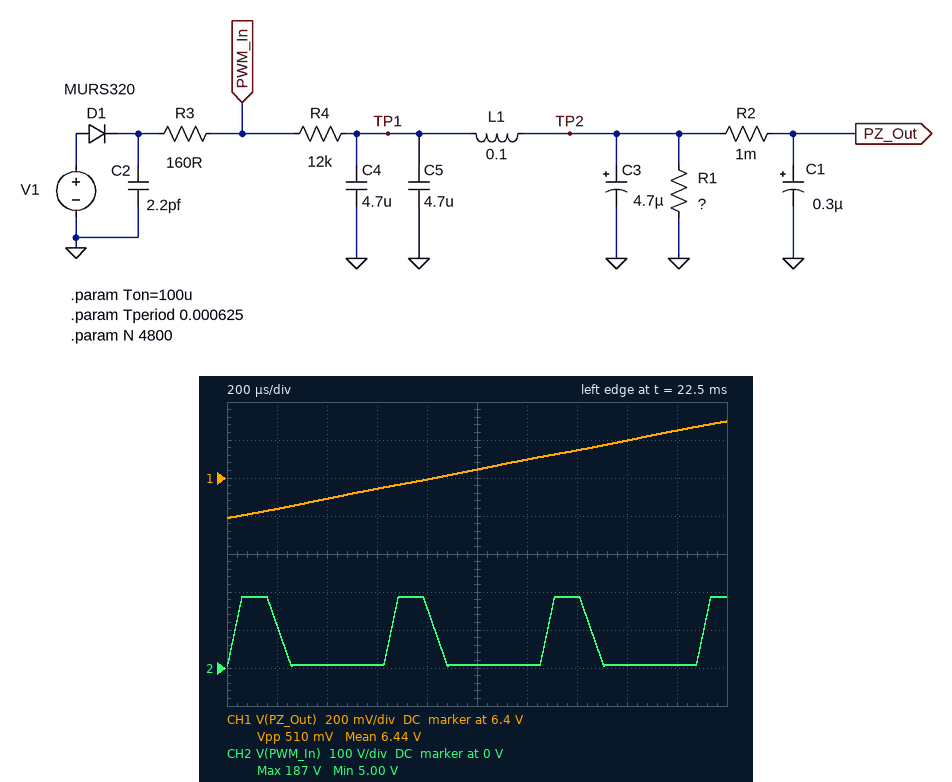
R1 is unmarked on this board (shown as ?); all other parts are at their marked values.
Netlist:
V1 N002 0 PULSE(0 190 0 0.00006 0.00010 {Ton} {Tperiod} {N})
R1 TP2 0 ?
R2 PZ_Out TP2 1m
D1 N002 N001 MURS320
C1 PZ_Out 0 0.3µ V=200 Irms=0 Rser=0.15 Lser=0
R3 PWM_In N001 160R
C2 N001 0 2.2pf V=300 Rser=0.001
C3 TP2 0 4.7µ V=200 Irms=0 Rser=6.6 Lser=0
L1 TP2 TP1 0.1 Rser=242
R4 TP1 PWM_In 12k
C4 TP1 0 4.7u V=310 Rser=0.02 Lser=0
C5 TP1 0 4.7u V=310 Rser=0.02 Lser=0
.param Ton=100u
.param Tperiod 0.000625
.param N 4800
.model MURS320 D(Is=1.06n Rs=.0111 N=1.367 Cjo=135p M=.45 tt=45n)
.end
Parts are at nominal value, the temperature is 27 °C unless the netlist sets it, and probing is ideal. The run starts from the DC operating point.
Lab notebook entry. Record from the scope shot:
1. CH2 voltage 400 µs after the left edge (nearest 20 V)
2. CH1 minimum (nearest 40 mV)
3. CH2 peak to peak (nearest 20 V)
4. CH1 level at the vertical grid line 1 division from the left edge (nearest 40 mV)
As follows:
0 V
6.20 V
180 V
6.24 V
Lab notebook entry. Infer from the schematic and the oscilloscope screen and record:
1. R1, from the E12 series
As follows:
12 kΩ
